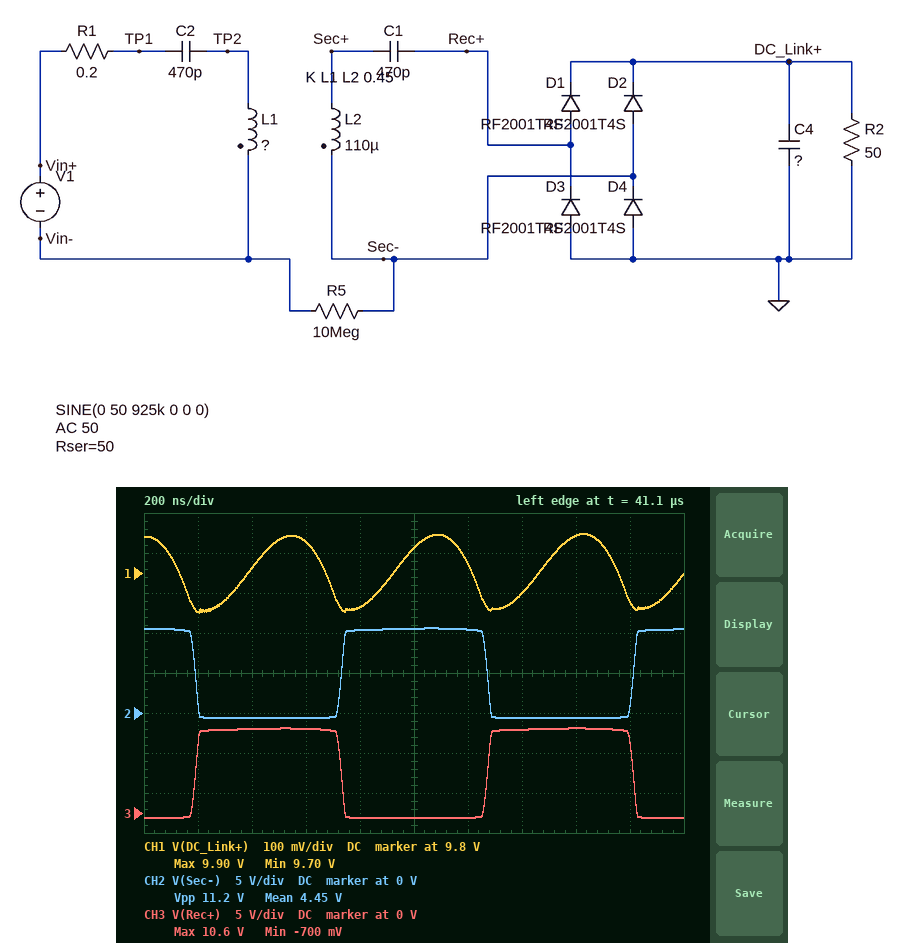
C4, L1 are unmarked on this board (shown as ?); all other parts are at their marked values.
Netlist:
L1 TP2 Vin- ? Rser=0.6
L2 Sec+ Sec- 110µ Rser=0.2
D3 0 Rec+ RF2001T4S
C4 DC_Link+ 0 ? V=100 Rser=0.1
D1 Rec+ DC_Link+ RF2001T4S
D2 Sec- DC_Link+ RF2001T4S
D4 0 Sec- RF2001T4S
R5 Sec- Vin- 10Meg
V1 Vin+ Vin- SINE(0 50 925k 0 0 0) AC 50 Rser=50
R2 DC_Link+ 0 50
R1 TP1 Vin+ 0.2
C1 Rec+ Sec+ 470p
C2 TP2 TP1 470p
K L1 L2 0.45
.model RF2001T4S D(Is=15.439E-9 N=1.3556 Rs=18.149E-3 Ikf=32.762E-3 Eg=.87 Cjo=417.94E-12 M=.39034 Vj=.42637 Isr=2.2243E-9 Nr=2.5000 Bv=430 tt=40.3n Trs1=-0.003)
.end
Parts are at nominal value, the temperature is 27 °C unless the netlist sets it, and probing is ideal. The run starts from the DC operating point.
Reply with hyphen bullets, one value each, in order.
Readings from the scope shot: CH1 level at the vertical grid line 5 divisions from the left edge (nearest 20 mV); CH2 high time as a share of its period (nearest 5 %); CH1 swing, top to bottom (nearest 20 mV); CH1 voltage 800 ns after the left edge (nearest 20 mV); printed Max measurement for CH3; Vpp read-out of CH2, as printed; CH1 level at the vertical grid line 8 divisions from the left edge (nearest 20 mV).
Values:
- 9.86 V
- 50 %
- 200 mV
- 9.72 V
- 10.6 V
- 11.2 V
- 9.90 V
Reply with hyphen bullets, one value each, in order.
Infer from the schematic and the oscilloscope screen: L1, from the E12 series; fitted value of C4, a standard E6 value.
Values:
- 180 µH
- 150 nF
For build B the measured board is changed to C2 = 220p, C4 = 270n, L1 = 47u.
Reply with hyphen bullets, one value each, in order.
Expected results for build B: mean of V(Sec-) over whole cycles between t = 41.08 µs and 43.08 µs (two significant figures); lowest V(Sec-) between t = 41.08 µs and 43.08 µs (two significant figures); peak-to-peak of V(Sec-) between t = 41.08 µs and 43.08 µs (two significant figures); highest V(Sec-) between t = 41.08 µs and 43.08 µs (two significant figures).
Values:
- 770 mV
- -570 mV
- 2.7 V
- 2.1 V
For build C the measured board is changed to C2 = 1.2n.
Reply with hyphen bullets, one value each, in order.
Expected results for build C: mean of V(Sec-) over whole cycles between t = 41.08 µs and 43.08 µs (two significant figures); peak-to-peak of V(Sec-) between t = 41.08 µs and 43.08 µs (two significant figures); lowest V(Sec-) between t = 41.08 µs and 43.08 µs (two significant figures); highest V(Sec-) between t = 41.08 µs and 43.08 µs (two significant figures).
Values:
- 2.5 V
- 6.4 V
- -640 mV
- 5.7 V
